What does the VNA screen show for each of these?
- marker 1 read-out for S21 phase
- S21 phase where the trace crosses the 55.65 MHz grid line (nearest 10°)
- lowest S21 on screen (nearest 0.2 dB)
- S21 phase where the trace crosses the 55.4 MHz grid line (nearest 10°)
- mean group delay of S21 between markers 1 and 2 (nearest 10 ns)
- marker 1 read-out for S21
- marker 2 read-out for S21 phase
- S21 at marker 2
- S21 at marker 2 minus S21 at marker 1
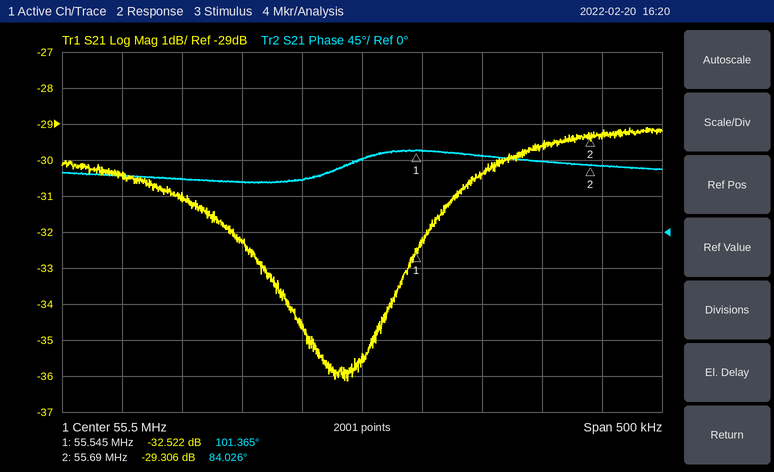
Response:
101.365°
90°
-36.2 dB
60°
330 ns
-32.522 dB
84.026°
-29.306 dB
3.216 dB
